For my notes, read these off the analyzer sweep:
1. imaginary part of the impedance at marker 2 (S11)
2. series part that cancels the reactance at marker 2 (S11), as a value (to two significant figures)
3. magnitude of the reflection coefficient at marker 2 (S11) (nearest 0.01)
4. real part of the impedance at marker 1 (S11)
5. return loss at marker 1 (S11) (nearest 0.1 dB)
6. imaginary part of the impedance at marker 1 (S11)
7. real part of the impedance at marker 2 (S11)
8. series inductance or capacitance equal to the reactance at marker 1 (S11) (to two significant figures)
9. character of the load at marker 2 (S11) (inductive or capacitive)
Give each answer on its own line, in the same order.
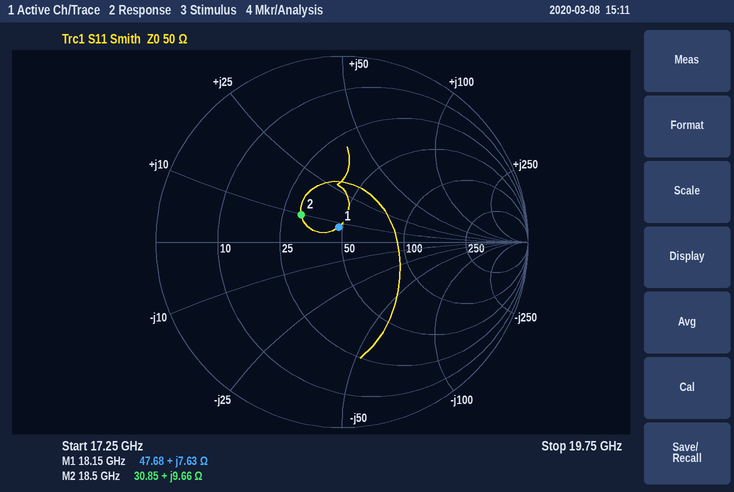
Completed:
+9.66 Ω
890 fF
0.26
47.68 Ω
21.8 dB
+7.63 Ω
30.85 Ω
67 pH
inductive
